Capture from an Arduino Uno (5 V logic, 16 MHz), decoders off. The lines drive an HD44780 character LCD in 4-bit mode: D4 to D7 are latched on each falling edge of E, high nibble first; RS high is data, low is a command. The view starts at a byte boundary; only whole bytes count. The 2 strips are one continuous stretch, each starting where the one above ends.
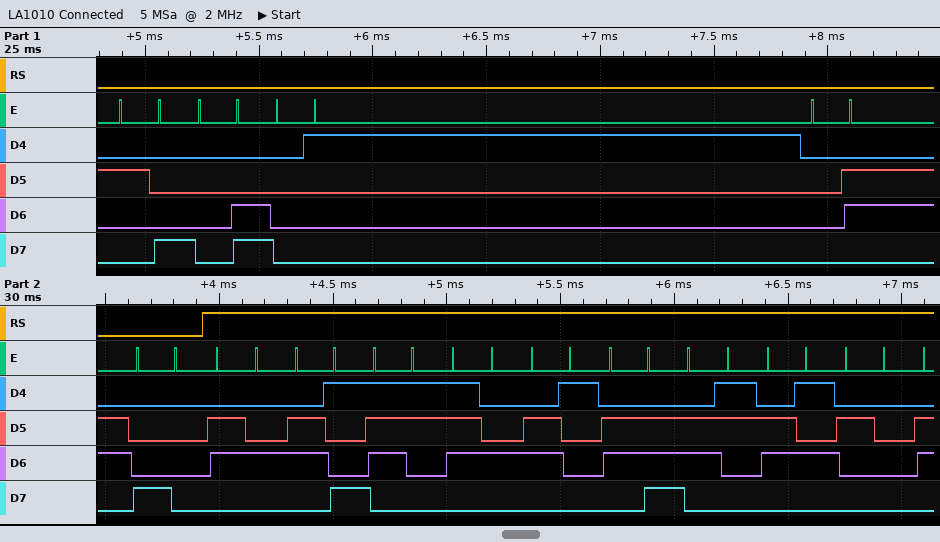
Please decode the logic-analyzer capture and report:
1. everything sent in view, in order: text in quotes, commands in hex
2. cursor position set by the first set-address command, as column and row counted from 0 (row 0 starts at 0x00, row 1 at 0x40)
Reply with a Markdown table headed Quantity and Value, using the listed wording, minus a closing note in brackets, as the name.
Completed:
| Quantity | Value |
|---|---|
| everything sent in view, in order: text in quotes, commands in hex | 0x28 0x0C 0x01 0x06 0x80 "distance " |
| cursor position set by the first set-address command, as column and row counted from 0 | column 0, row 0 |
